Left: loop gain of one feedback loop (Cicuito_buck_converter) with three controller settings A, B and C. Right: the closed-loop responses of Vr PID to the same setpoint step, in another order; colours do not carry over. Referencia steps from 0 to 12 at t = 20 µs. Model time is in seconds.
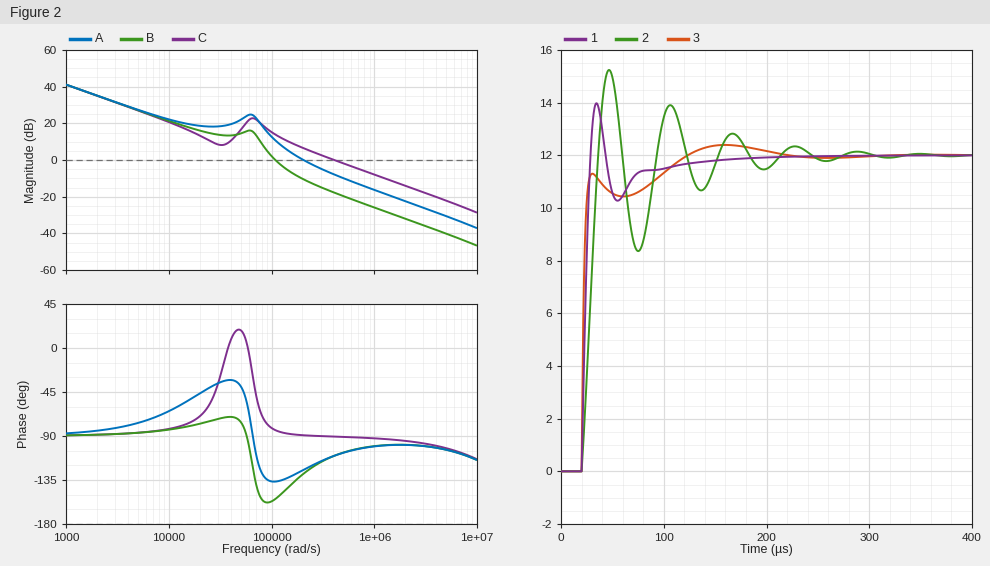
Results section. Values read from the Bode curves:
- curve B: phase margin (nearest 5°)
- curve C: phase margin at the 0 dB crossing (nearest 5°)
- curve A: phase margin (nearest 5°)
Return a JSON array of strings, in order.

["25°", "90°", "55°"]
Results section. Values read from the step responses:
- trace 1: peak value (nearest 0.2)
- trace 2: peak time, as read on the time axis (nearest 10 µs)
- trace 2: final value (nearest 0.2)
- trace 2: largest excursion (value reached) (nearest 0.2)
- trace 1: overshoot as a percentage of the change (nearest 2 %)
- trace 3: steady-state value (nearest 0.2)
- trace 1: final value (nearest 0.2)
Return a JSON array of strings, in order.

["14.0", "50 µs", "12.0", "15.2", "16 %", "12.0", "12.0"]
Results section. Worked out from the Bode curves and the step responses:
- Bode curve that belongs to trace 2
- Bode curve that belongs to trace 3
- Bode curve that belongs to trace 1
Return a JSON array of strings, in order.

["B", "C", "A"]
